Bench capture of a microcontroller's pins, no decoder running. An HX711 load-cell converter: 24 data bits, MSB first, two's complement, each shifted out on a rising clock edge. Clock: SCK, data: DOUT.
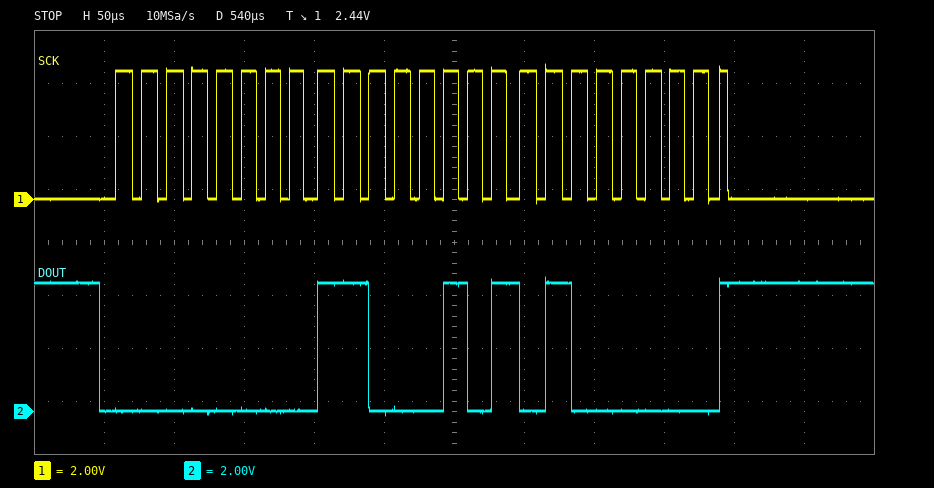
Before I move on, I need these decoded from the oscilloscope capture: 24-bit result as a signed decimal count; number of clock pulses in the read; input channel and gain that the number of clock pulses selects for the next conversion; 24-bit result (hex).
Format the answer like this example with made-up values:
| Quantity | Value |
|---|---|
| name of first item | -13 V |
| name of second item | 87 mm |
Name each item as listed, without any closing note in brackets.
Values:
| Quantity | Value |
|---|---|
| 24-bit result as a signed decimal count | 50496 |
| number of clock pulses in the read | 25 |
| input channel and gain that the number of clock pulses selects for the next conversion | channel A, gain 128 |
| 24-bit result | 0x00C540 |
